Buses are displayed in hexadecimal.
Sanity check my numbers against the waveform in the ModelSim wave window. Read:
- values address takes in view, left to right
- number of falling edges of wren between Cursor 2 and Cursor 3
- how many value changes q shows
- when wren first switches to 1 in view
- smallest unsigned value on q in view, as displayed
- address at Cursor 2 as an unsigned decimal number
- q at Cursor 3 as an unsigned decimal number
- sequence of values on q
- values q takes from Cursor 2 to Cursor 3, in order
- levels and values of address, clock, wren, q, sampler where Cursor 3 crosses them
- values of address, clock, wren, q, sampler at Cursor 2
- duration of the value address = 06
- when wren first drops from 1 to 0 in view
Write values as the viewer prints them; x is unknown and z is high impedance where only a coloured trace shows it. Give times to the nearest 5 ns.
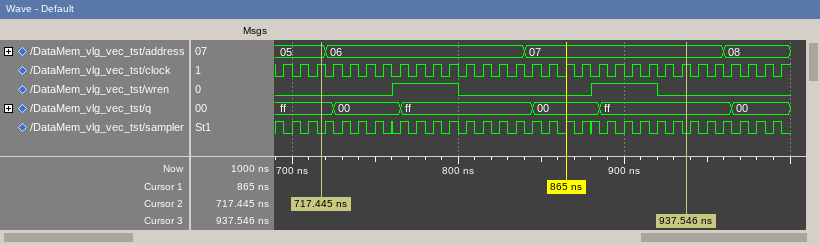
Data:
05, 06, 07, 08
2
5
760 ns
00
5
255
ff, 00, ff, 00, ff, 00
ff, 00, ff, 00, ff
address=07, clock=1, wren=0, q=ff, sampler=0
address=05, clock=1, wren=0, q=ff, sampler=0
120 ns
800 ns
